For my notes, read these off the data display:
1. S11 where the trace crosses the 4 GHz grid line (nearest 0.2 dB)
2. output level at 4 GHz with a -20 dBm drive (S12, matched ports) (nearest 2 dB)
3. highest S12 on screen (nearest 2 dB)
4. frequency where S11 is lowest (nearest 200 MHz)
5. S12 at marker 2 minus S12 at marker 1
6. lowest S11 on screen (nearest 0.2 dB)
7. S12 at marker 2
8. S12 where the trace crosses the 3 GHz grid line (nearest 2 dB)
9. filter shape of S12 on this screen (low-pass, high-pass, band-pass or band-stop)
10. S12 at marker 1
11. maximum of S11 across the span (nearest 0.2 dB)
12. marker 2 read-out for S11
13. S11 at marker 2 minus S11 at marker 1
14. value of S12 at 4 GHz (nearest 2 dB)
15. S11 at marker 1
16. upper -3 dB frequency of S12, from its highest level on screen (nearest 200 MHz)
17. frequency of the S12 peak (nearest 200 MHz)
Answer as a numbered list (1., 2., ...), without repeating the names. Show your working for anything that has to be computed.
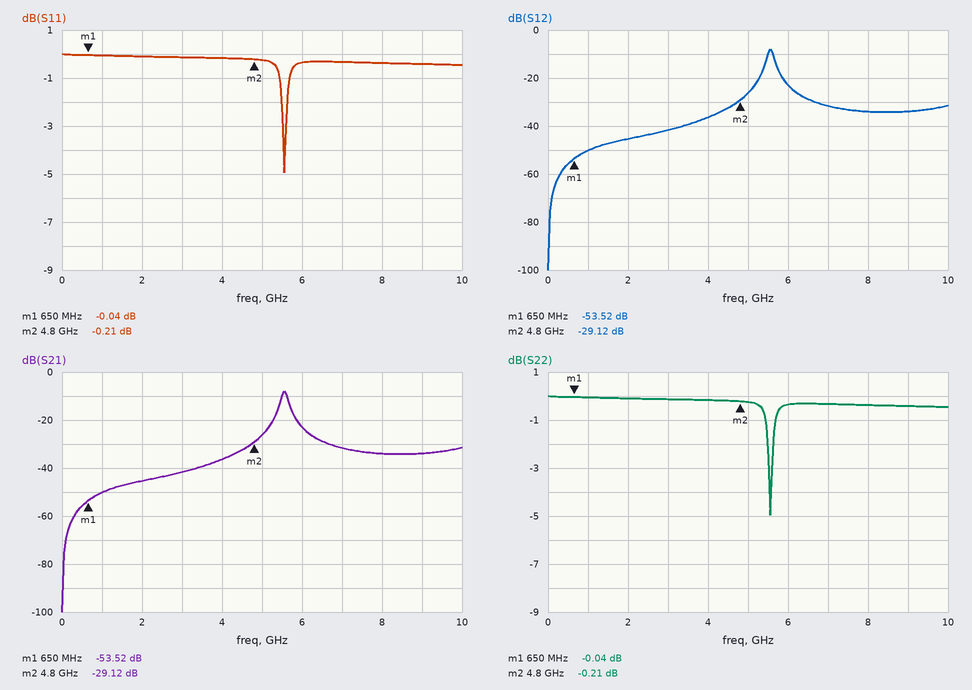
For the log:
1. -0.2 dB
2. -20 dBm + (-36 dB) = -56 dBm
3. -8 dB
4. 5.6 GHz
5. -29.12 − (-53.52) = 24.40 dB
6. -5.0 dB
7. -29.12 dB
8. -42 dB
9. band-pass
10. -53.52 dB
11. 0.0 dB
12. -0.21 dB
13. -0.21 − (-0.04) = -0.17 dB
14. -36 dB
15. -0.04 dB
16. 5.6 GHz
17. 5.6 GHz
